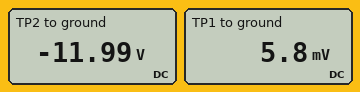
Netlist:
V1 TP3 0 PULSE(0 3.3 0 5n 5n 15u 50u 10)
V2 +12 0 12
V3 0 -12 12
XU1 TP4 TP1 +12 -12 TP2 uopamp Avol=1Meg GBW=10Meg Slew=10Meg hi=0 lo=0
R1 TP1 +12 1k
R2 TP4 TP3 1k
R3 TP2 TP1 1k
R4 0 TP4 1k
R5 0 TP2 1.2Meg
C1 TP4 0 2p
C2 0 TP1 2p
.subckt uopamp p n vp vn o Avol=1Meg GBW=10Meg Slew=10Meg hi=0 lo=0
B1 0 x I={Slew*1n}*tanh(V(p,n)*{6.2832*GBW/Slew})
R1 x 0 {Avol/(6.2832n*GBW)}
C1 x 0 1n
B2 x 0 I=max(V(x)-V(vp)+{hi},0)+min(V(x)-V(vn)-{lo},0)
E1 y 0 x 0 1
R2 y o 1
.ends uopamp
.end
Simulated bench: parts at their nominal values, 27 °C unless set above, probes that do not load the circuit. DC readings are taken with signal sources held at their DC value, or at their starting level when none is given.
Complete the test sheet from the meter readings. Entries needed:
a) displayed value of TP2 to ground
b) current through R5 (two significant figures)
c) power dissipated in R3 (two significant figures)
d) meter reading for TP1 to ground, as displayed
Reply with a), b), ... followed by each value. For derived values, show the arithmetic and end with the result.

a) -11.99 V
b) (0 V - (-11.99 V)) / 1.2 MΩ = 10 µA
c) (5.8 mV - (-11.99 V))^2 / 1 kΩ = 140 mW
d) 5.8 mV
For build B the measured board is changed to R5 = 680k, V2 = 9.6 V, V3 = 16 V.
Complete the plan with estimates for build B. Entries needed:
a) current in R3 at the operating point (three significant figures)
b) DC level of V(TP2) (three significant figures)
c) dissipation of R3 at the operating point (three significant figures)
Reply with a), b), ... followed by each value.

a) 9.60 mA
b) -9.60 V
c) 92.2 mW
